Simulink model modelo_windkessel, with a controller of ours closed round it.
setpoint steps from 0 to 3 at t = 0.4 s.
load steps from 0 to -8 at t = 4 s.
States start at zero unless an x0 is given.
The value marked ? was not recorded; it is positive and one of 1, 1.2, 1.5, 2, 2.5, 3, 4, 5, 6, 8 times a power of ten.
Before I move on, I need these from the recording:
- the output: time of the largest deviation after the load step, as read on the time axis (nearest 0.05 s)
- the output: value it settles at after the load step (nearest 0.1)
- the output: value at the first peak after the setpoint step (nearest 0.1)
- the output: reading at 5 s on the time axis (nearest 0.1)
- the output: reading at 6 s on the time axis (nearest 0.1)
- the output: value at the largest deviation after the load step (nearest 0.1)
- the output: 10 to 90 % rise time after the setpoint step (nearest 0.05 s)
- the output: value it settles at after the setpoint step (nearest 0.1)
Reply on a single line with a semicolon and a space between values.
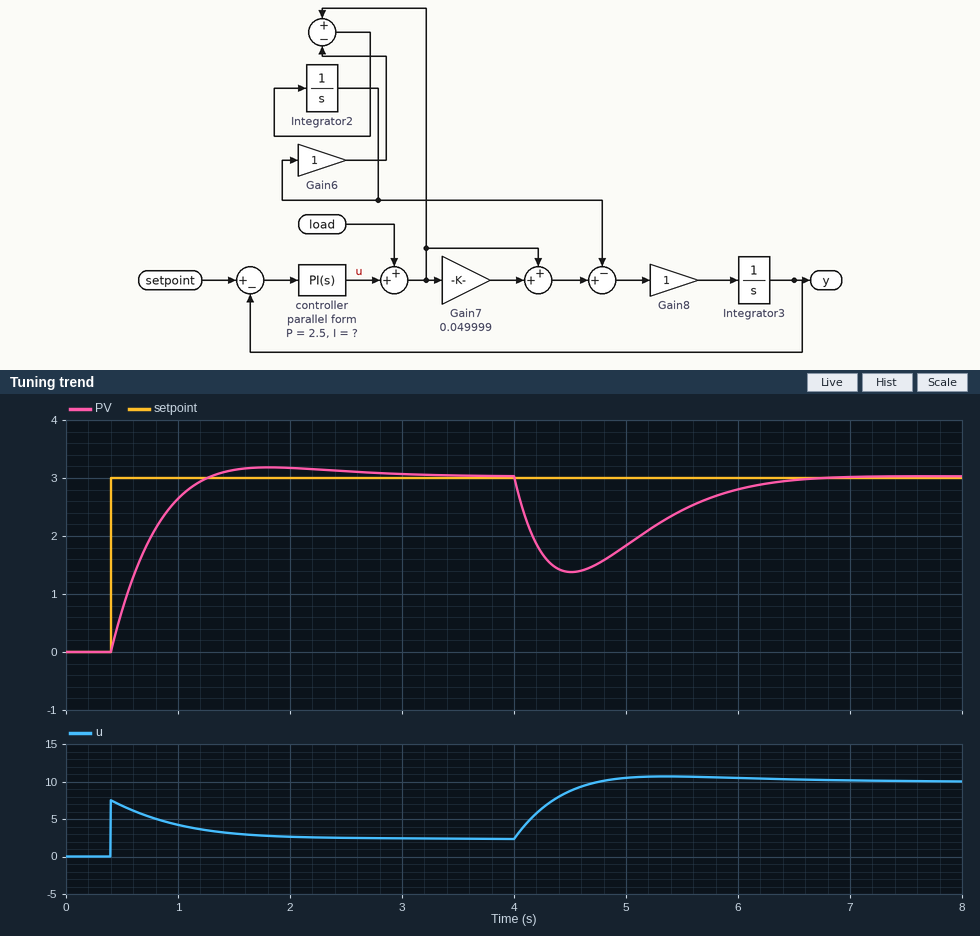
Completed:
4.50 s; 3.0; 3.2; 1.8; 2.8; 1.4; 0.60 s; 3.0
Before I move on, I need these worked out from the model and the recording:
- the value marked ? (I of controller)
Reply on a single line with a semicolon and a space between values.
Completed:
4
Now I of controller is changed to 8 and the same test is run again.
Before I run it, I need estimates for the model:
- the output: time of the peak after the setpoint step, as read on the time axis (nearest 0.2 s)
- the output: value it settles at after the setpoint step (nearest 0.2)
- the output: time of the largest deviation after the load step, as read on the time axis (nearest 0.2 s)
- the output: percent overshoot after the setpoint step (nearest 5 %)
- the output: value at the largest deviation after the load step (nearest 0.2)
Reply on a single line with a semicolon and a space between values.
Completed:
1.4 s; 3.0; 4.4 s; 15 %; 1.6
